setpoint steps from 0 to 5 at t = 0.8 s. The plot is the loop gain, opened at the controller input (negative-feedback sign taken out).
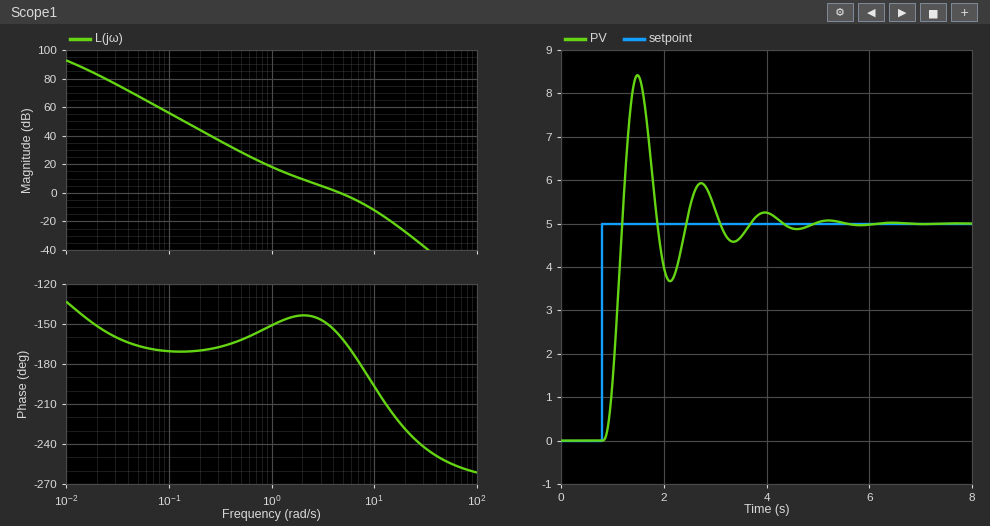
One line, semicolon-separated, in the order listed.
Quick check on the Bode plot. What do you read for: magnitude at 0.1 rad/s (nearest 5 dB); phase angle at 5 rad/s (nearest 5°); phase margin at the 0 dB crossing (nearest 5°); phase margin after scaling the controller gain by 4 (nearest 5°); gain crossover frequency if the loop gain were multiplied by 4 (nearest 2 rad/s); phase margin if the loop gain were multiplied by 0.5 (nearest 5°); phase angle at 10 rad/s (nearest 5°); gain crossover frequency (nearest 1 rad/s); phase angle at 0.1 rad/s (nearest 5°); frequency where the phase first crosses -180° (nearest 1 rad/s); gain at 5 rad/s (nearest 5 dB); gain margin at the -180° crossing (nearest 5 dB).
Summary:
55 dB; -160°; 20°; -15°; 10 rad/s; 35°; -195°; 5 rad/s; -170°; 7 rad/s; 0 dB; 5 dB
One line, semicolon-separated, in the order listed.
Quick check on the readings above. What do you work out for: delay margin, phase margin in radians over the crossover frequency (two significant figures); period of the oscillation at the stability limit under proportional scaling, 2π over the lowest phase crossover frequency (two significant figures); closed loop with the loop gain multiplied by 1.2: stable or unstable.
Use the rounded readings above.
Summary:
0.070 s; 0.90 s; stable
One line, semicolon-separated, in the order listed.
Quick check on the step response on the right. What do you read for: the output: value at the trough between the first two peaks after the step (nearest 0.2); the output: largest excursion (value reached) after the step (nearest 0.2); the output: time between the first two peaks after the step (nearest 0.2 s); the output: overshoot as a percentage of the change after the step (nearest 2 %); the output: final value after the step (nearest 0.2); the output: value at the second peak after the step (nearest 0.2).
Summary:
3.6; 8.4; 1.2 s; 68 %; 5.0; 6.0
